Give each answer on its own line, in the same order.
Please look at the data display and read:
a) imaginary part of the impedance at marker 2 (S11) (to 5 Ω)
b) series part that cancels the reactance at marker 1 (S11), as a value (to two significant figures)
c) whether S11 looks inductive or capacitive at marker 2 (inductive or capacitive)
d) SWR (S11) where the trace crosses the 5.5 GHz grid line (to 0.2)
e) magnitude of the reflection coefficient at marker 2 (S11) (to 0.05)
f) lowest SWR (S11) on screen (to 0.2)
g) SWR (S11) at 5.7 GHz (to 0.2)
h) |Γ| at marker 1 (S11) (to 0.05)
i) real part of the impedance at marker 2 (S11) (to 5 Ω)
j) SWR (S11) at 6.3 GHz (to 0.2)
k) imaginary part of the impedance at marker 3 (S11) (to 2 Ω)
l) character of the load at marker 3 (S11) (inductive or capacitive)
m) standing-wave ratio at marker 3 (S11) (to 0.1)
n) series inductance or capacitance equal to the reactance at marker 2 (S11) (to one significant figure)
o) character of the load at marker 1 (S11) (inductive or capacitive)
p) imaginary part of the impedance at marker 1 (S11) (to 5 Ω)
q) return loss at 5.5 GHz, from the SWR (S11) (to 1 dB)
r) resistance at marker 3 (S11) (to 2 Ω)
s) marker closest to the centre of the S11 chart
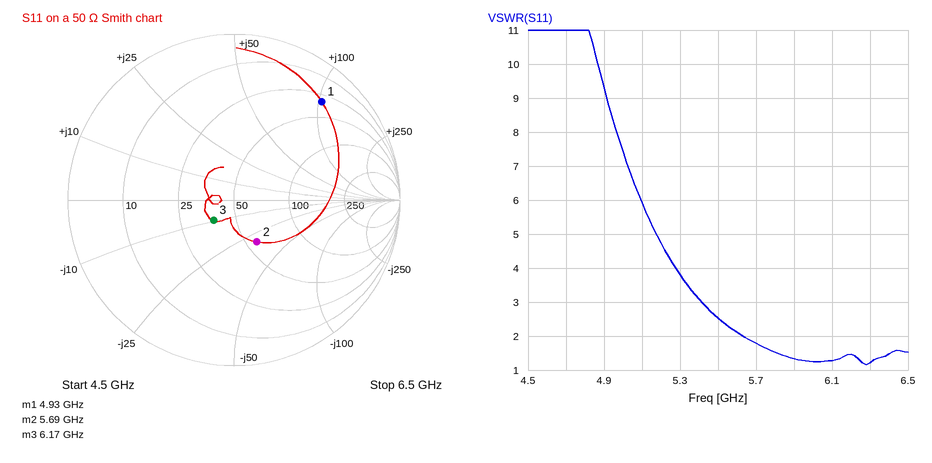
-30 Ω
310 fF
capacitive
2.6
0.30
1.2
1.8
0.80
55 Ω
1.2
-10 Ω
capacitive
1.4
900 fF
inductive
+105 Ω
7 dB
38 Ω
marker 3
